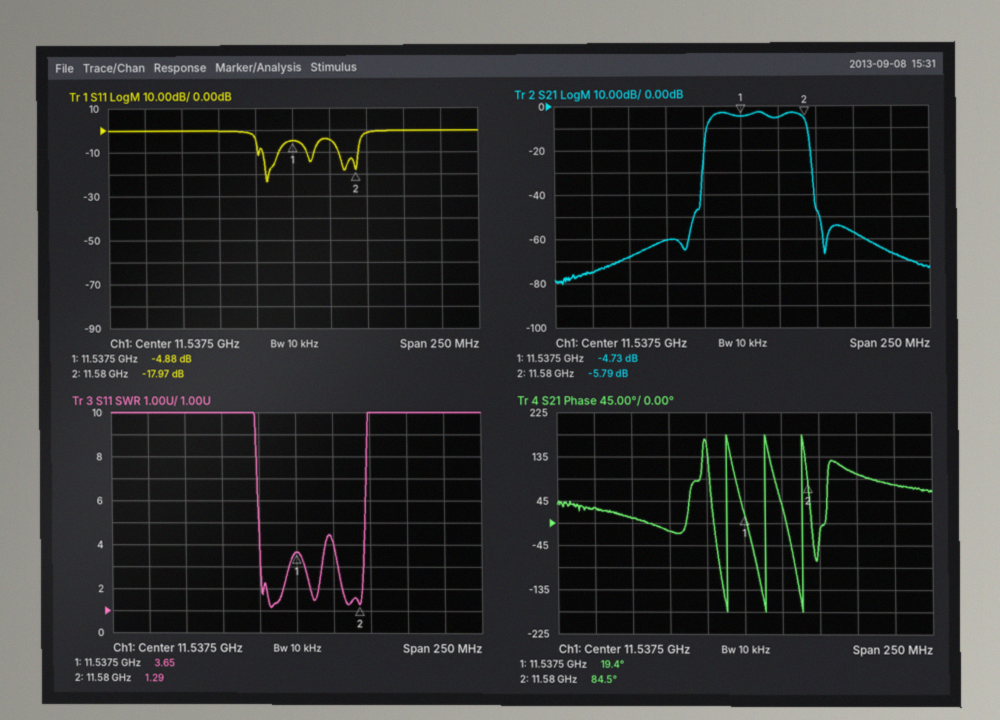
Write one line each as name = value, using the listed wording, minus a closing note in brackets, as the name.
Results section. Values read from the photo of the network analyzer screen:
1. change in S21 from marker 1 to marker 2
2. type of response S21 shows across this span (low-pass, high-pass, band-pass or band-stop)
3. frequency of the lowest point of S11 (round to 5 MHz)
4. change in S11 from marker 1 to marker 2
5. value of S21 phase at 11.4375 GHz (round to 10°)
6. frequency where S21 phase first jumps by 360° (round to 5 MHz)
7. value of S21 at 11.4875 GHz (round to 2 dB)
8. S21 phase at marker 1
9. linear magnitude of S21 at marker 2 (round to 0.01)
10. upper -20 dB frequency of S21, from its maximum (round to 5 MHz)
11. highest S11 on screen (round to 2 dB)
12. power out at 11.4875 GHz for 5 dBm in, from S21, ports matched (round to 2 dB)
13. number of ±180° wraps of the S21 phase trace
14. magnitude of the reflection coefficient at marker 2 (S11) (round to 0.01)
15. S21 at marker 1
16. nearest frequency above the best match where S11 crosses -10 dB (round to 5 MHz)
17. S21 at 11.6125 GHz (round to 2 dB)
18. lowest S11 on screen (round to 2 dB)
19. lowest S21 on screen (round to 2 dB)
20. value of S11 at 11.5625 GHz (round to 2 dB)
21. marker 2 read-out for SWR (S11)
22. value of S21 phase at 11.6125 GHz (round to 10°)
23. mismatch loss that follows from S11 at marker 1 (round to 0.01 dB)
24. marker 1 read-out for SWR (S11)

change in S21 from marker 1 to marker 2 = -1.06 dB
type of response S21 shows across this span = band-pass
frequency of the lowest point of S11 = 11.520 GHz
change in S11 from marker 1 to marker 2 = -13.09 dB
value of S21 phase at 11.4375 GHz = 30°
frequency where S21 phase first jumps by 360° = 11.525 GHz
value of S21 at 11.4875 GHz = -60 dB
S21 phase at marker 1 = 19.4°
linear magnitude of S21 at marker 2 = 0.51
upper -20 dB frequency of S21, from its maximum = 11.585 GHz
highest S11 on screen = 0 dB
power out at 11.4875 GHz for 5 dBm in, from S21, ports matched = -56 dBm
number of ±180° wraps of the S21 phase trace = 3
magnitude of the reflection coefficient at marker 2 (S11) = 0.13
S21 at marker 1 = -4.73 dB
nearest frequency above the best match where S11 crosses -10 dB = 11.530 GHz
S21 at 11.6125 GHz = -58 dB
lowest S11 on screen = -24 dB
lowest S21 on screen = -80 dB
value of S11 at 11.5625 GHz = -4 dB
marker 2 read-out for SWR = 1.29
value of S21 phase at 11.6125 GHz = 100°
mismatch loss that follows from S11 at marker 1 = 1.71 dB
marker 1 read-out for SWR = 3.65
